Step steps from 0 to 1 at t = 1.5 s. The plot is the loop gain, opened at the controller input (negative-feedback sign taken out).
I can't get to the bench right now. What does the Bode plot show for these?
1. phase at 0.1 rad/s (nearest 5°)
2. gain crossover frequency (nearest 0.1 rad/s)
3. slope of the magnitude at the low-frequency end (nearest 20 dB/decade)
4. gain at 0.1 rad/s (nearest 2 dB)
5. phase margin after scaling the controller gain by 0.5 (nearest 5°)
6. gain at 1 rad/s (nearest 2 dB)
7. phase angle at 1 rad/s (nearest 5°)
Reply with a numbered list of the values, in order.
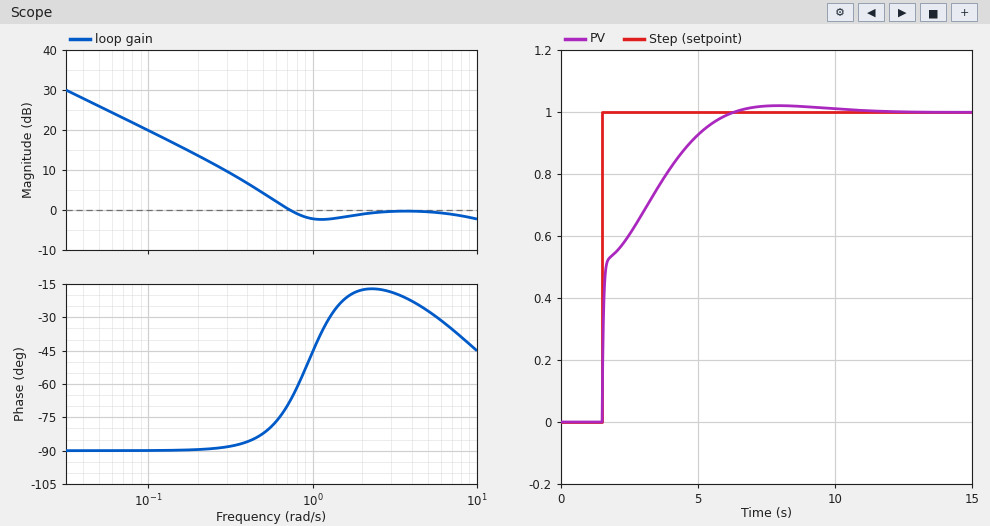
1. -90°
2. 0.7 rad/s
3. -20 dB/decade
4. 20 dB
5. 95°
6. -2 dB
7. -45°
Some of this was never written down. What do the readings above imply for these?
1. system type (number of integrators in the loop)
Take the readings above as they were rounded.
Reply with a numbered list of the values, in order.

1. 1
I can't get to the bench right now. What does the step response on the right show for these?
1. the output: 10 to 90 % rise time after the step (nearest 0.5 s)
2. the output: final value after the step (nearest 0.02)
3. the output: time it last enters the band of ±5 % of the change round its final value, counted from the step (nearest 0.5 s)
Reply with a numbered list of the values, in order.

1. 3.0 s
2. 1.00
3. 4.0 s
